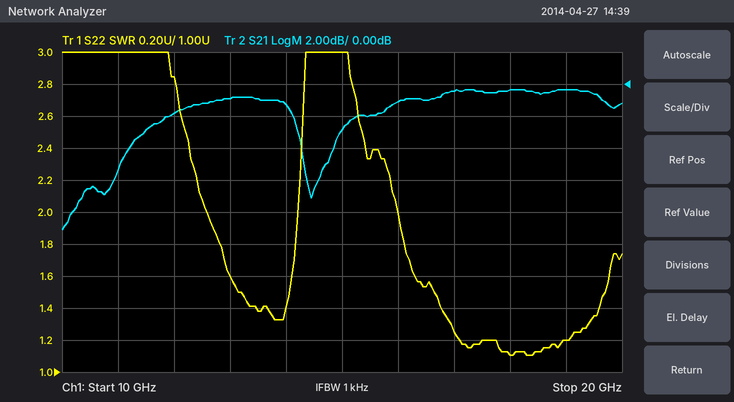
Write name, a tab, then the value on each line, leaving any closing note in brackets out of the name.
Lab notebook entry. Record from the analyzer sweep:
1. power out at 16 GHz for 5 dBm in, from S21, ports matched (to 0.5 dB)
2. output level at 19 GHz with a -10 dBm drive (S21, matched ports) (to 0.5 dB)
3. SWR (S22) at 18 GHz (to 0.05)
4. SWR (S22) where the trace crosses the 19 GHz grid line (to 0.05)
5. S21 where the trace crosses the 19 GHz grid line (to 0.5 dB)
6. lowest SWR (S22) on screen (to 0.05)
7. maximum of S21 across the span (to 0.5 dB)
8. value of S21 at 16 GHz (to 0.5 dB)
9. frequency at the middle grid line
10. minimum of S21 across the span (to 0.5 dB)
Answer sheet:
power out at 16 GHz for 5 dBm in, from S21, ports matched	4.0 dBm
output level at 19 GHz with a -10 dBm drive (S21, matched ports)	-10.5 dBm
SWR (S22) at 18 GHz	1.10
SWR (S22) where the trace crosses the 19 GHz grid line	1.20
S21 where the trace crosses the 19 GHz grid line	-0.5 dB
lowest SWR (S22) on screen	1.10
maximum of S21 across the span	-0.5 dB
value of S21 at 16 GHz	-1.0 dB
frequency at the middle grid line	15 GHz
minimum of S21 across the span	-9.0 dB
